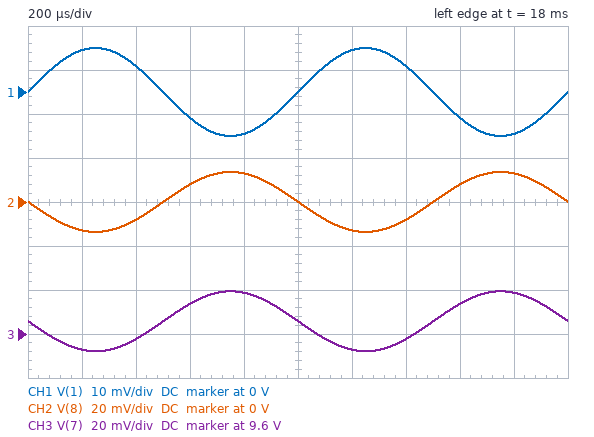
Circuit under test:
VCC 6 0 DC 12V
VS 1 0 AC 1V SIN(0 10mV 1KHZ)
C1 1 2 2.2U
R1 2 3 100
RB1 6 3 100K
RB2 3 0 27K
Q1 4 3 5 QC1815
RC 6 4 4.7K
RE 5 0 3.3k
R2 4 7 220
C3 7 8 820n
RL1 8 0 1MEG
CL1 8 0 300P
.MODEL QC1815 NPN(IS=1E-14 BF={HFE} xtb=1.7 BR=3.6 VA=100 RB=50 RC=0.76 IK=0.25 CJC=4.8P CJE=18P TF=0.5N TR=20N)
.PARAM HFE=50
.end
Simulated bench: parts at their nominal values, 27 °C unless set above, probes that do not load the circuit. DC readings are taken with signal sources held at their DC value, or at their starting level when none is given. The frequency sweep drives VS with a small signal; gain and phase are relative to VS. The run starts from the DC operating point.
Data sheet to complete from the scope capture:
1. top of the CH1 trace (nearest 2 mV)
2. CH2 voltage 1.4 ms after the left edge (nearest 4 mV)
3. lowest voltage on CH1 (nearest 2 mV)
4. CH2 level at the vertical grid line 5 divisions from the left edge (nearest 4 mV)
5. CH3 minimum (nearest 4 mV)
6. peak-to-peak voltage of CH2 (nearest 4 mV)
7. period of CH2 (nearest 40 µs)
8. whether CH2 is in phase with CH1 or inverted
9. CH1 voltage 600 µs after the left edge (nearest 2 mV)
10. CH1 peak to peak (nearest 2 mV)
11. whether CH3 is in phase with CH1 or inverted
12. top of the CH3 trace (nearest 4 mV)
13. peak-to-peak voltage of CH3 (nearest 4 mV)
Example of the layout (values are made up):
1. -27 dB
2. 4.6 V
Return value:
1. 10 mV
2. -8 mV
3. -10 mV
4. 0 V
5. 9.592 V
6. 28 mV
7. 1.00 ms
8. inverted
9. -6 mV
10. 20 mV
11. inverted
12. 9.620 V
13. 28 mV
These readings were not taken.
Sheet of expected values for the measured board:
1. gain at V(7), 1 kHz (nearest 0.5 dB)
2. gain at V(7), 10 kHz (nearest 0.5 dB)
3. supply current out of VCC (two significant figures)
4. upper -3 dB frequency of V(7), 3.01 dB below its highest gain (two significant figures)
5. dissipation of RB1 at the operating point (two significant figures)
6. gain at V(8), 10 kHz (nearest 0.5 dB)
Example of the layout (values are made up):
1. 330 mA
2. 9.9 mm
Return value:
1. 2.5 dB
2. 2.5 dB
3. 610 µA
4. 110 kHz
5. 930 µW
6. 2.5 dB
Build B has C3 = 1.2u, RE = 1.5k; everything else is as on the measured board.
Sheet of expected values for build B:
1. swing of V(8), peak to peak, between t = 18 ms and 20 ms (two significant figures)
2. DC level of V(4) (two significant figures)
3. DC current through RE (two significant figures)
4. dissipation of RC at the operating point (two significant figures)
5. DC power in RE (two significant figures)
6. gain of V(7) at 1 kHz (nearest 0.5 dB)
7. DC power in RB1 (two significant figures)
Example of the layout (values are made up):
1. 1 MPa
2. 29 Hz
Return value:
1. 60 mV
2. 7.4 V
3. 1.0 mA
4. 4.5 mW
5. 1.5 mW
6. 9.5 dB
7. 970 µW
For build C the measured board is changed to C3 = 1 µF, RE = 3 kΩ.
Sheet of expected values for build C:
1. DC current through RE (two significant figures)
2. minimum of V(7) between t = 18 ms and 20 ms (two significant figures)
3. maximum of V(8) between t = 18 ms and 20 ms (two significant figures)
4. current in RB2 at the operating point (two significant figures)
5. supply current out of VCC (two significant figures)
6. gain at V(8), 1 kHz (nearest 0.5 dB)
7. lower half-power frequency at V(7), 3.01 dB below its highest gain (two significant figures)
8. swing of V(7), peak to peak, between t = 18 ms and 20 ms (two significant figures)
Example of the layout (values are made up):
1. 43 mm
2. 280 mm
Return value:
1. 560 µA
2. 9.4 V
3. 15 mV
4. 86 µA
5. 650 µA
6. 3.5 dB
7. 3.8 Hz
8. 30 mV
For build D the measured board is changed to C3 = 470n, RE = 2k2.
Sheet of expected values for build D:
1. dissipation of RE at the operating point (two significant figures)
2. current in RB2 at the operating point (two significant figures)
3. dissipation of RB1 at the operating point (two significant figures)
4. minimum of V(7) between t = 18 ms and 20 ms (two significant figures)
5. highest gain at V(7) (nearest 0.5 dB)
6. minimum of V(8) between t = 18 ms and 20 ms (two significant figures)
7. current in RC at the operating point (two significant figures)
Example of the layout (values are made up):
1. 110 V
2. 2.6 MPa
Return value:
1. 1.2 mW
2. 84 µA
3. 950 µW
4. 8.6 V
5. 6.0 dB
6. -20 mV
7. 720 µA
